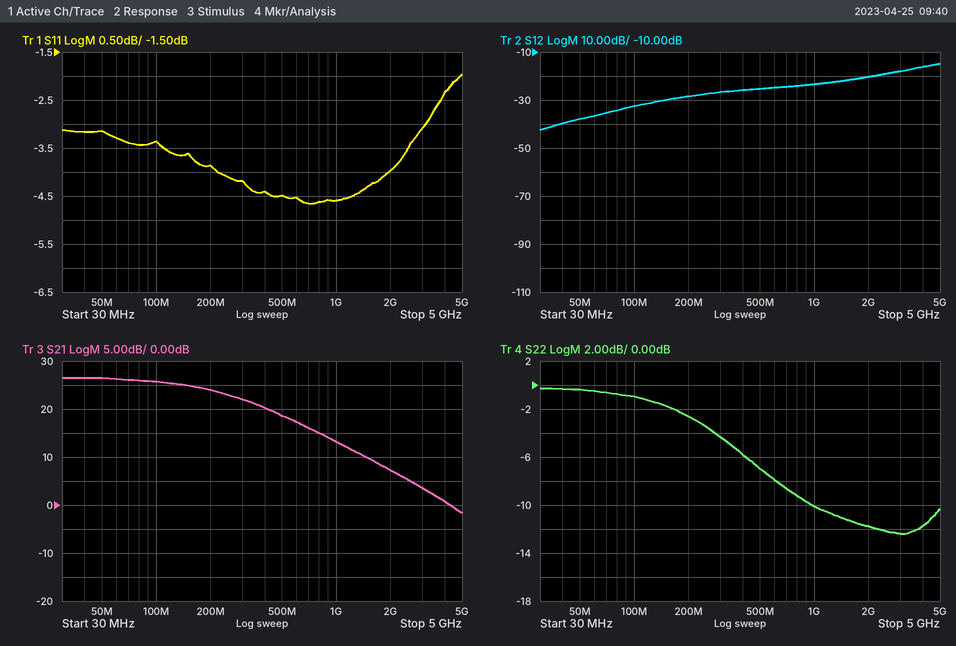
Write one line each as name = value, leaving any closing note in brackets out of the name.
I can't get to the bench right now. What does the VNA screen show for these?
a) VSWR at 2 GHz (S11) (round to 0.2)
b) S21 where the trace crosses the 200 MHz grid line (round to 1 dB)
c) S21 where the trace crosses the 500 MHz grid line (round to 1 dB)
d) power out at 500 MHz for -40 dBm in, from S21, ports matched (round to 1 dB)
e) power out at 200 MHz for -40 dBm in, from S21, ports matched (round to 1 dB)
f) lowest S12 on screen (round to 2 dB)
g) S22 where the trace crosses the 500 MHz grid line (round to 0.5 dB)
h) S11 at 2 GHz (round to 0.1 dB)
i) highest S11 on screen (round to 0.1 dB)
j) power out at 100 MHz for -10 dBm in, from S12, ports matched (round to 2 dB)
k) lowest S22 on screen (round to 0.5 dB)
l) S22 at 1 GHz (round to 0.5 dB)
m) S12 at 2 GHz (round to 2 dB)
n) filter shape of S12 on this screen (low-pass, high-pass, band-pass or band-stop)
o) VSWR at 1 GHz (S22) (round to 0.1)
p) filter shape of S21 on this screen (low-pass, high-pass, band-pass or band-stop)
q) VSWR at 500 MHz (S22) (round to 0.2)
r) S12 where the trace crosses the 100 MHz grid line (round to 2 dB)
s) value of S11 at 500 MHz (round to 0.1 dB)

VSWR at 2 GHz (S11) = 4.4
S21 where the trace crosses the 200 MHz grid line = 24 dB
S21 where the trace crosses the 500 MHz grid line = 19 dB
power out at 500 MHz for -40 dBm in, from S21, ports matched = -21 dBm
power out at 200 MHz for -40 dBm in, from S21, ports matched = -16 dBm
lowest S12 on screen = -42 dB
S22 where the trace crosses the 500 MHz grid line = -7.0 dB
S11 at 2 GHz = -4.0 dB
highest S11 on screen = -2.0 dB
power out at 100 MHz for -10 dBm in, from S12, ports matched = -42 dBm
lowest S22 on screen = -12.5 dB
S22 at 1 GHz = -10.0 dB
S12 at 2 GHz = -20 dB
filter shape of S12 on this screen = high-pass
VSWR at 1 GHz (S22) = 1.9
filter shape of S21 on this screen = low-pass
VSWR at 500 MHz (S22) = 2.6
S12 where the trace crosses the 100 MHz grid line = -32 dB
value of S11 at 500 MHz = -4.5 dB
